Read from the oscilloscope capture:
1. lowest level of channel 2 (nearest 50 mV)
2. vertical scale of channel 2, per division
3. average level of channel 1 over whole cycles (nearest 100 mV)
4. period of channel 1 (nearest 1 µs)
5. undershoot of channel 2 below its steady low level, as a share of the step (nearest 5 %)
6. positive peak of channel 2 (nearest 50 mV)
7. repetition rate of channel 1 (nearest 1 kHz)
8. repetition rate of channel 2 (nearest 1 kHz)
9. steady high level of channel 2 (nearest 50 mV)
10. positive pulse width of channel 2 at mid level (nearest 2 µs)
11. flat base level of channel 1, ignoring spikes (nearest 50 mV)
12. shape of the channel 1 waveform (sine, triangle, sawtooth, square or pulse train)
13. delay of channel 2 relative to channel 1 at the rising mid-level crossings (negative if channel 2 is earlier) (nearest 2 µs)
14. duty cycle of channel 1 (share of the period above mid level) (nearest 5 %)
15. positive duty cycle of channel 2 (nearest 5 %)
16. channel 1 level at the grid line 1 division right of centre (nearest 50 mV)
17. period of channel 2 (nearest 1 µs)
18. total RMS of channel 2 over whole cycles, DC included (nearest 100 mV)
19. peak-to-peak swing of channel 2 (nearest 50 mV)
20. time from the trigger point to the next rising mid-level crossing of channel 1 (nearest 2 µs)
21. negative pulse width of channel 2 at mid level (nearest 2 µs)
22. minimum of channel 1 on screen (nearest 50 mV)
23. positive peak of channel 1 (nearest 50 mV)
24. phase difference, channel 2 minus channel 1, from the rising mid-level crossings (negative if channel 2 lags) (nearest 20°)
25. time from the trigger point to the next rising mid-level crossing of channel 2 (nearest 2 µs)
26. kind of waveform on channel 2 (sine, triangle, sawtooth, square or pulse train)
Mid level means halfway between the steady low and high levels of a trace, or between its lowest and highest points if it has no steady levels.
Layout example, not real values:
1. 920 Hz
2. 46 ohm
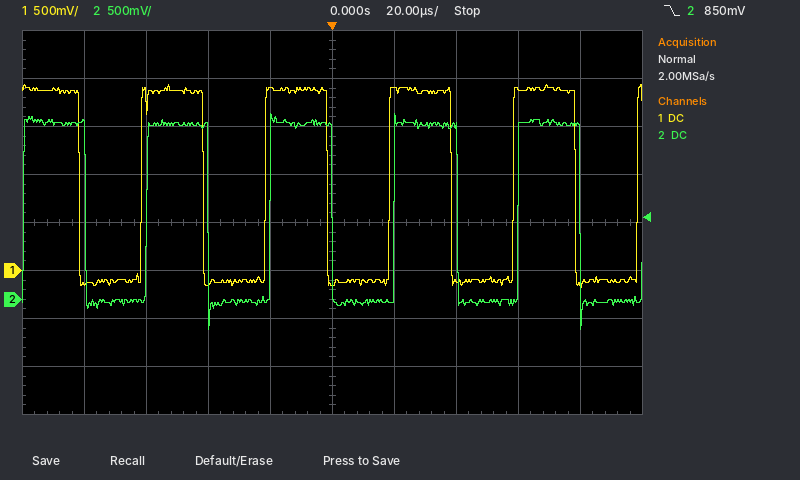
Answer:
1. -300 mV
2. 500 mV
3. 900 mV
4. 40 µs
5. 15 %
6. 1.95 V
7. 25 kHz
8. 25 kHz
9. 1.85 V
10. 20 µs
11. -100 mV
12. square
13. +2 µs
14. 50 %
15. 50 %
16. 1.90 V
17. 40 µs
18. 1.3 V
19. 2.25 V
20. 18 µs
21. 20 µs
22. -200 mV
23. 1.95 V
24. -20°
25. 20 µs
26. square
